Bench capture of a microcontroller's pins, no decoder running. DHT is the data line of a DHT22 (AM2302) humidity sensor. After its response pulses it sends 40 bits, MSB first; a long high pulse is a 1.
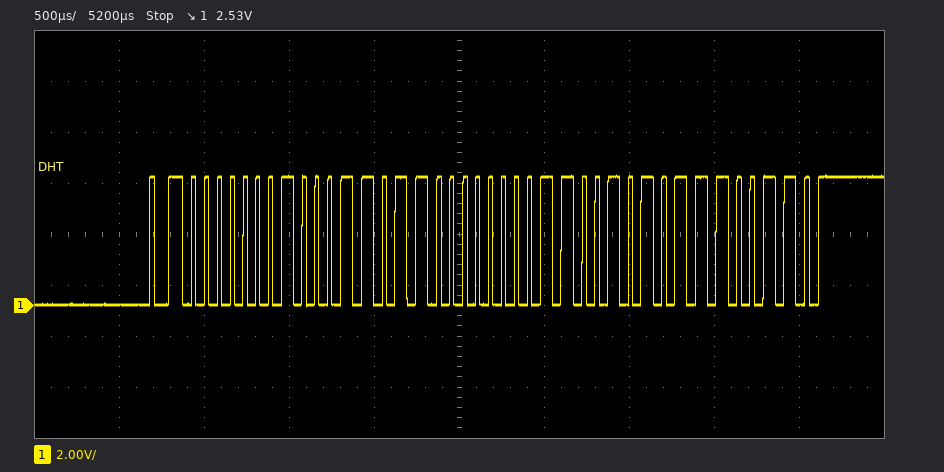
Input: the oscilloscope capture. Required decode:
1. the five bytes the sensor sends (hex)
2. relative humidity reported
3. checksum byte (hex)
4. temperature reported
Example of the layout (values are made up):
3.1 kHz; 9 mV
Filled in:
01 1B 00 CA E6; 28.3 %; 0xE6; 20.2 °C
